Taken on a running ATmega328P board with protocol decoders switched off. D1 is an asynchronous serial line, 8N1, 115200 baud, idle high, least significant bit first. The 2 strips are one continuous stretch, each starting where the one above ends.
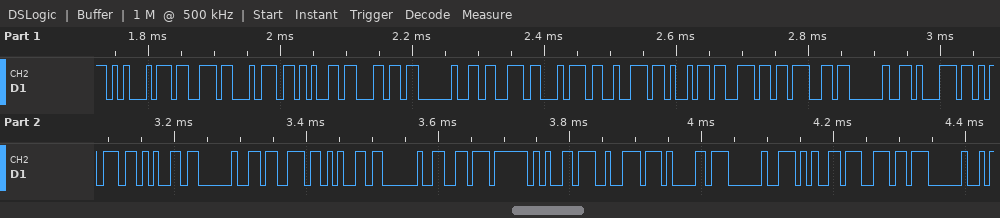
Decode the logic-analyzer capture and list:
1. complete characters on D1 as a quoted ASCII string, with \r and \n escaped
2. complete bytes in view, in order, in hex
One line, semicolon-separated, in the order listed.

"Estel string que se vera en "; 45 73 74 65 6C 20 73 74 72 69 6E 67 20 71 75 65 20 73 65 20 76 65 72 61 20 65 6E 20
